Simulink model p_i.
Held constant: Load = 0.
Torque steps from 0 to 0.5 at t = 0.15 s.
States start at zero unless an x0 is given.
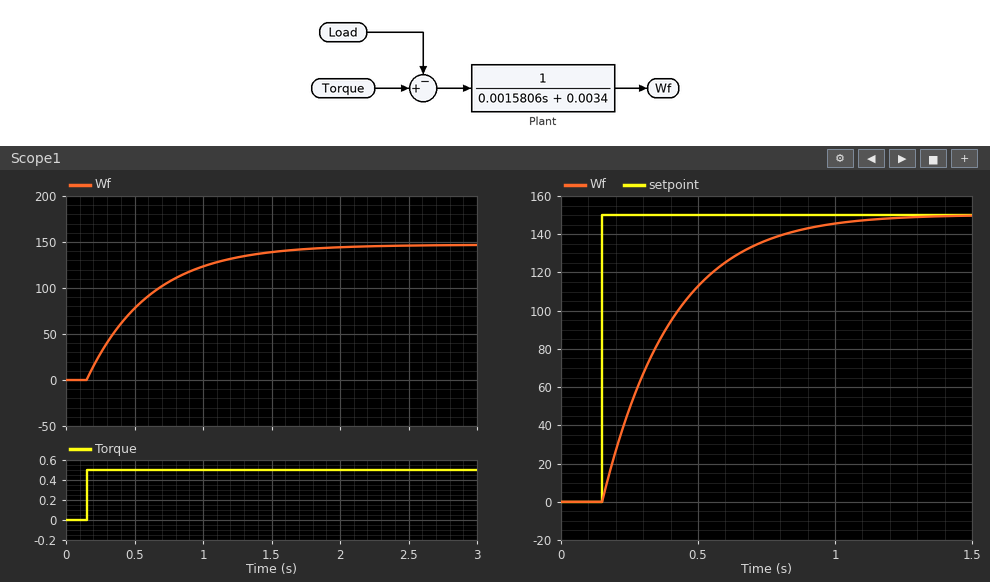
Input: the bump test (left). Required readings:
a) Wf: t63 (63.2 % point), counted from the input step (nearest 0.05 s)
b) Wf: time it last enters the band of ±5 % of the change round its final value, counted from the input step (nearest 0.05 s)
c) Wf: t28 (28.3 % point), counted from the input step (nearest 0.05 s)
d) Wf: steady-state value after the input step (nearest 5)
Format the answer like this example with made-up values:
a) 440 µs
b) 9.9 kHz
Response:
a) 0.45 s
b) 1.40 s
c) 0.15 s
d) 145
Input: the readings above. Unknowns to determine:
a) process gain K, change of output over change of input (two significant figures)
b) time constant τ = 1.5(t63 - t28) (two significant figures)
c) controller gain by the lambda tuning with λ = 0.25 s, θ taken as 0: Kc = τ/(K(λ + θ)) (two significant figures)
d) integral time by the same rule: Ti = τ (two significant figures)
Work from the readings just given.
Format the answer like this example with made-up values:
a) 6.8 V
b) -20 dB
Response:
a) 290
b) 0.45 s
c) 0.0062
d) 0.45 s
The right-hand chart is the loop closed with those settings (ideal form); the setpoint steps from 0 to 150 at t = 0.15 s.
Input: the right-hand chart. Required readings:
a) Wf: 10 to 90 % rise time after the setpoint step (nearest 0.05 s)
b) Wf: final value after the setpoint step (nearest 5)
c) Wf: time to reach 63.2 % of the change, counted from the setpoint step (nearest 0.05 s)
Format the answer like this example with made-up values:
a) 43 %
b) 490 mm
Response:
a) 0.55 s
b) 150
c) 0.25 s
